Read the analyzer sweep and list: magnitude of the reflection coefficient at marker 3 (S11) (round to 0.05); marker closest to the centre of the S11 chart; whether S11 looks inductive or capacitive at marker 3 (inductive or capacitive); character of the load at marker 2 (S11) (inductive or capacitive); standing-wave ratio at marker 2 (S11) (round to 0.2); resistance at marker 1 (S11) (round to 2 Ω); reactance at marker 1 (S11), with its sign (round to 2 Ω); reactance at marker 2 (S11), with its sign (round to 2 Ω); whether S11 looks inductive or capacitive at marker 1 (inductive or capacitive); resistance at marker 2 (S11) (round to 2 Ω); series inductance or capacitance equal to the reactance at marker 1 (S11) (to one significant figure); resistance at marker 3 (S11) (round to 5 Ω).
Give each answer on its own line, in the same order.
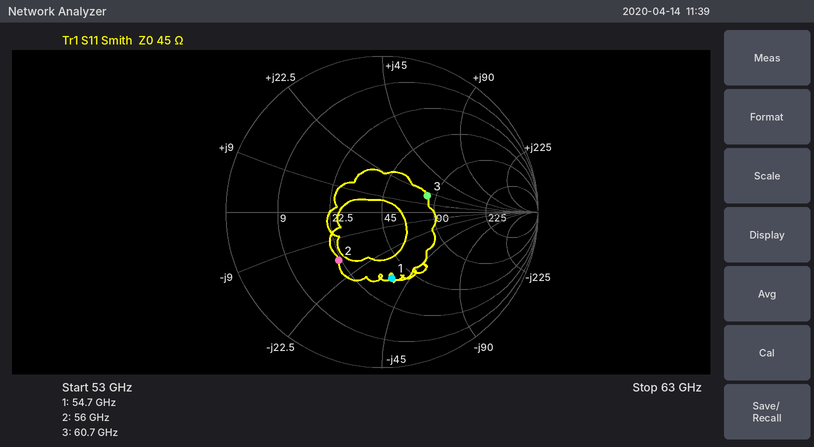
0.30
marker 3
inductive
capacitive
2.4
34 Ω
-36 Ω
-16 Ω
capacitive
22 Ω
80 fF
80 Ω
